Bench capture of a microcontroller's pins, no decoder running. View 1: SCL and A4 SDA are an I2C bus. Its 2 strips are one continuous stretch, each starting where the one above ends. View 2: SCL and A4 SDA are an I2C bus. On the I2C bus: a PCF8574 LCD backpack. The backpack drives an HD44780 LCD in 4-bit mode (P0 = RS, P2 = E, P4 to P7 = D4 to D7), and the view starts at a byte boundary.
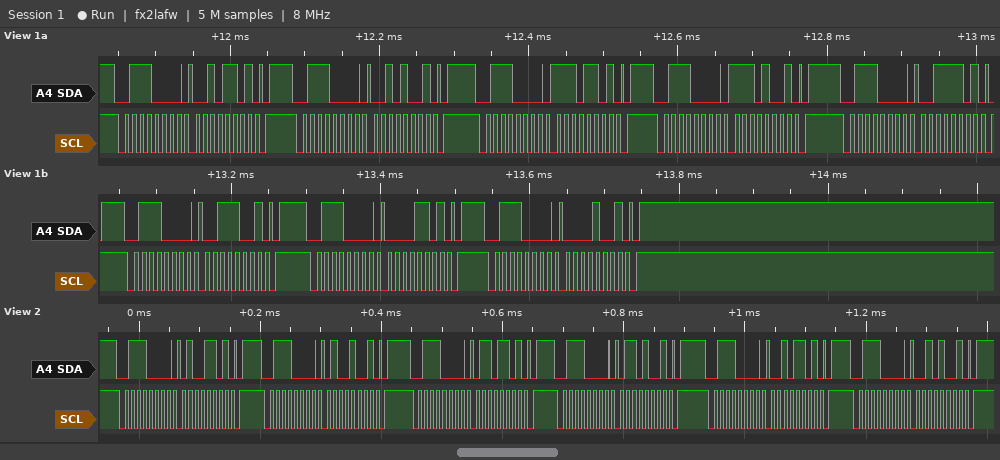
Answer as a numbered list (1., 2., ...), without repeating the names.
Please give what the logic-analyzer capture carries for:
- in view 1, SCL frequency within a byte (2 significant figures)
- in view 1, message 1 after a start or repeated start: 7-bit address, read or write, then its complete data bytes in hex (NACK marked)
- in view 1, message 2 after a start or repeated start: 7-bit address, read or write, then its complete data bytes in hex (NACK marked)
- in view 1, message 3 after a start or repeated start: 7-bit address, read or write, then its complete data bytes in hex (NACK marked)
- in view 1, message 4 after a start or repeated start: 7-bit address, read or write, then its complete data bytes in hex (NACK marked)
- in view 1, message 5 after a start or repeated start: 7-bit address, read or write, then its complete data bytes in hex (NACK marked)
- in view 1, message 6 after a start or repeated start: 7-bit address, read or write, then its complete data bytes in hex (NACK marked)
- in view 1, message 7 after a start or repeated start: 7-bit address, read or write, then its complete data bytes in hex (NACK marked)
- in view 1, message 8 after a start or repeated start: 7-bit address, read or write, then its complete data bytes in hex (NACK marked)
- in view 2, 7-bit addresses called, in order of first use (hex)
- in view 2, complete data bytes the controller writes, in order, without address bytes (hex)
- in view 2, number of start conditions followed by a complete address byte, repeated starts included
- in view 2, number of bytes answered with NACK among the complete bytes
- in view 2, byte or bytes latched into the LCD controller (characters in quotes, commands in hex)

1. 100 kHz
2. 0x38 write: 2D
3. 0x38 write: 29
4. 0x38 write: ED
5. 0x38 write: E9
6. 0x38 write: 3D
7. 0x38 write: 39
8. 0x38 write: 0D
9. 0x38 write: 09
10. 0x38
11. 4D 49 6D 69 2D 29
12. 6
13. 0
14. 'F'
